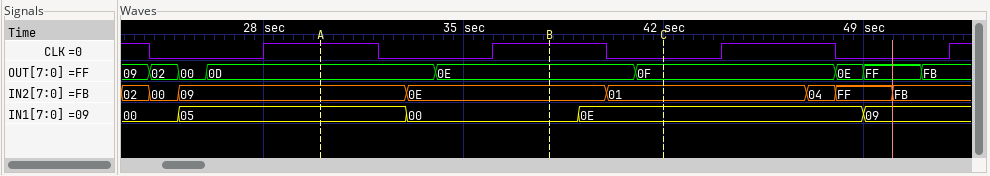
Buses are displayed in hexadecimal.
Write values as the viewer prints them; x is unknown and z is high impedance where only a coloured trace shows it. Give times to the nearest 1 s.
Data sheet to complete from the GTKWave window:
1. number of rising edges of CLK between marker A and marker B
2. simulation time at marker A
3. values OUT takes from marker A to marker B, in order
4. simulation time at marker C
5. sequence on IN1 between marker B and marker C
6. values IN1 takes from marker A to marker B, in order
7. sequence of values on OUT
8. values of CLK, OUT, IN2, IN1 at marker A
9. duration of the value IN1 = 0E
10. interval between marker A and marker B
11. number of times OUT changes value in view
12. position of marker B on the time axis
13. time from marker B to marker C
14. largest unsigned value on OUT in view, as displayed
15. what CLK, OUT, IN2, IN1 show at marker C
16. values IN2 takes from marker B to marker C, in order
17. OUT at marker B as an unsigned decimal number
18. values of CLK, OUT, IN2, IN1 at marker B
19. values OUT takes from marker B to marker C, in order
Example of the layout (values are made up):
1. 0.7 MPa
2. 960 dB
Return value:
1. 1
2. 30 s
3. 0D, 0E
4. 42 s
5. 00, 0E
6. 05, 00
7. 09, 02, 00, 0D, 0E, 0F, 0E, FF, FB
8. CLK=1, OUT=0D, IN2=09, IN1=05
9. 10 s
10. 8 s
11. 8
12. 38 s
13. 4 s
14. FF
15. CLK=0, OUT=0F, IN2=01, IN1=0E
16. 0E, 01
17. 14
18. CLK=1, OUT=0E, IN2=0E, IN1=00
19. 0E, 0F
